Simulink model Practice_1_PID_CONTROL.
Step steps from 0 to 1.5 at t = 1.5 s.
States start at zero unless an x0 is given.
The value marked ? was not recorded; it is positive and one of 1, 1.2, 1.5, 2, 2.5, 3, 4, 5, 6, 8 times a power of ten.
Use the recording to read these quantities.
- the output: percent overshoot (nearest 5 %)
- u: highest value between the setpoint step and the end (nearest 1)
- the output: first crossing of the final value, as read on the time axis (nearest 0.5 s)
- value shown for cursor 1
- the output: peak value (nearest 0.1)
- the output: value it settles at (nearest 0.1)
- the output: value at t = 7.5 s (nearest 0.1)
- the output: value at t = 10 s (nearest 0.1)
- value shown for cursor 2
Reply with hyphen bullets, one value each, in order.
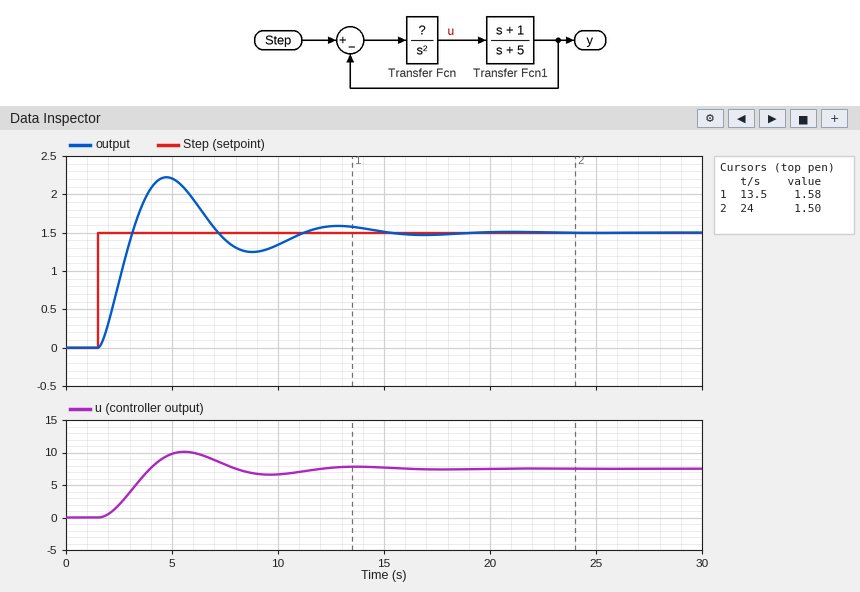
- 50 %
- 10
- 3.0 s
- 1.58
- 2.2
- 1.5
- 1.4
- 1.3
- 1.50
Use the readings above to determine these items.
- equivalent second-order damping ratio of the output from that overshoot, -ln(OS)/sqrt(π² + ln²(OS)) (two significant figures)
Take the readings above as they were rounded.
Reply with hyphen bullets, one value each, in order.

- 0.22
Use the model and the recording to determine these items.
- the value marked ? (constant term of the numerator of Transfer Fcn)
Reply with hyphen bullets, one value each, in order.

- 3
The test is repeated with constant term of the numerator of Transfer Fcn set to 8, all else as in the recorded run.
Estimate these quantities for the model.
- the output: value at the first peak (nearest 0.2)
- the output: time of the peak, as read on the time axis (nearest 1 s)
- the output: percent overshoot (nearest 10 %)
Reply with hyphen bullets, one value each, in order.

- 2.0
- 3 s
- 40 %
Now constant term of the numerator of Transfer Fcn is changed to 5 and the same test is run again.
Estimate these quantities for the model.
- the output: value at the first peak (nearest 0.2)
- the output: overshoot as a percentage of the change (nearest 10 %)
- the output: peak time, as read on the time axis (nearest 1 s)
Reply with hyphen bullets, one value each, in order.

- 2.2
- 40 %
- 4 s
